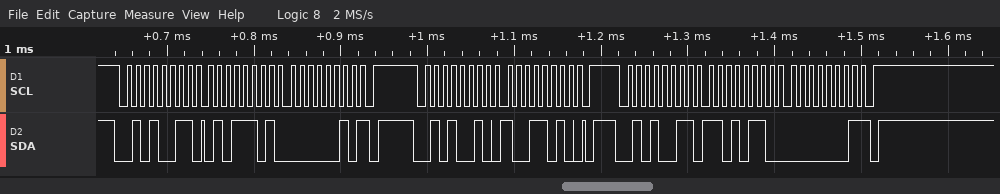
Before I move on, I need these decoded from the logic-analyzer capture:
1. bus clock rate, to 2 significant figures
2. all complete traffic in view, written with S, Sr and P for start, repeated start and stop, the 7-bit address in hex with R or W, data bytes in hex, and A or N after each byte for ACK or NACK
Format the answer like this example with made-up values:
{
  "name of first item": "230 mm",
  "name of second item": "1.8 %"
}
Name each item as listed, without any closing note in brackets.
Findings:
{
  "bus clock rate, to 2 significant figures": "100 kHz",
  "all complete traffic in view, written with S, Sr and P for start, repeated start and stop, the 7-bit address in hex with R or W, data bytes in hex, and A or N after each byte for ACK or NACK": "S 29R A 5D A 02 N P S 29W A 9A A P S 29R A D6 A 01 N P"
}
